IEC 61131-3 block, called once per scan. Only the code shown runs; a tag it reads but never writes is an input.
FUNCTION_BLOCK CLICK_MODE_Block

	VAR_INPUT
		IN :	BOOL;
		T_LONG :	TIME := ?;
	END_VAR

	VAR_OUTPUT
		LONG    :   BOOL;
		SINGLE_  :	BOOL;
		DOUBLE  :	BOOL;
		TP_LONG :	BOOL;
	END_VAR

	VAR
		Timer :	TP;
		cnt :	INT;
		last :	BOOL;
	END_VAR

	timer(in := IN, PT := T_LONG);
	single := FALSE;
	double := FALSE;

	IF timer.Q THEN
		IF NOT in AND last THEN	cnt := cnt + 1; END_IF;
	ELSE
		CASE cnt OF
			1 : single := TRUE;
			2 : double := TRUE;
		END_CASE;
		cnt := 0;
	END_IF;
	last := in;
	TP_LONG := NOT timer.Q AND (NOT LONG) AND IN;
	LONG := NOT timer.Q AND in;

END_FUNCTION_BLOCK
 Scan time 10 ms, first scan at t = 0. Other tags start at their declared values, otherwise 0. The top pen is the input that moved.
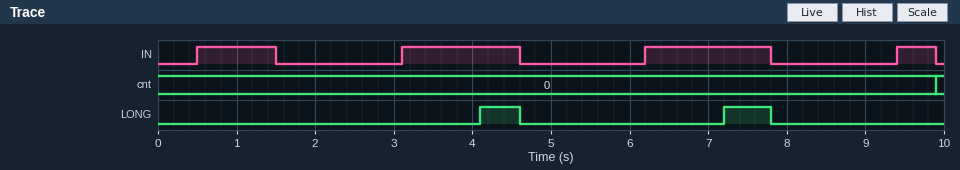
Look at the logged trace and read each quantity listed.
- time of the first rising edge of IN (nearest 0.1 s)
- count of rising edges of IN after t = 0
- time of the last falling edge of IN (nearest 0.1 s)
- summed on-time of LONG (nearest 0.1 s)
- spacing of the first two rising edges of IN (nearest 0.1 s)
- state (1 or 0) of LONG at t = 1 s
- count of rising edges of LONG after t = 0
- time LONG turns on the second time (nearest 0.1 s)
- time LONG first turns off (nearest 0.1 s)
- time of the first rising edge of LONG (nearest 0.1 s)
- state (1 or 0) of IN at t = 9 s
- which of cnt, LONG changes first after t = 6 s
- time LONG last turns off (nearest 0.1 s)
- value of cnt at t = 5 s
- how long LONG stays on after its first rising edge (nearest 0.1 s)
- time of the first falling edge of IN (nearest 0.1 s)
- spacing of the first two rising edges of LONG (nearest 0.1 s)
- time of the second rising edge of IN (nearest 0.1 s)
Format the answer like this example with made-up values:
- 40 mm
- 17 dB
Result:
- 0.5 s
- 4
- 9.9 s
- 1.1 s
- 2.6 s
- 0
- 2
- 7.2 s
- 4.6 s
- 4.1 s
- 0
- LONG
- 7.8 s
- 0
- 0.5 s
- 1.5 s
- 3.1 s
- 3.1 s
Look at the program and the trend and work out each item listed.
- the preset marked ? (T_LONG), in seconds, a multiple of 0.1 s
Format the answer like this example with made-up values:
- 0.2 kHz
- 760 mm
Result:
- 1.0 s
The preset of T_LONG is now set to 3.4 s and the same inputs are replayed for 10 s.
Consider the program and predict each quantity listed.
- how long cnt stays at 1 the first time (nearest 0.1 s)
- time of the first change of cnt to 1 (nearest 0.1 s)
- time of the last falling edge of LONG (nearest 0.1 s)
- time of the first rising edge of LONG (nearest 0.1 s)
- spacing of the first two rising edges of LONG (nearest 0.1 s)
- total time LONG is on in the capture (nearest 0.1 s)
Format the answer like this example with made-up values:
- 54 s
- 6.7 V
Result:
- 2.4 s
- 1.5 s
- 9.9 s
- 3.9 s
- 5.7 s
- 1.0 s
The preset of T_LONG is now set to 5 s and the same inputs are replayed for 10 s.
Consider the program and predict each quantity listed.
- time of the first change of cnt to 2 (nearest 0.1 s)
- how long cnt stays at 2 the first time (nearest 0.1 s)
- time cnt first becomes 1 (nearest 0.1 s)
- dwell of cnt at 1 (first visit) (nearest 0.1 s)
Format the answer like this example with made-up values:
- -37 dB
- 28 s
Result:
- 4.6 s
- 0.9 s
- 1.5 s
- 3.1 s
